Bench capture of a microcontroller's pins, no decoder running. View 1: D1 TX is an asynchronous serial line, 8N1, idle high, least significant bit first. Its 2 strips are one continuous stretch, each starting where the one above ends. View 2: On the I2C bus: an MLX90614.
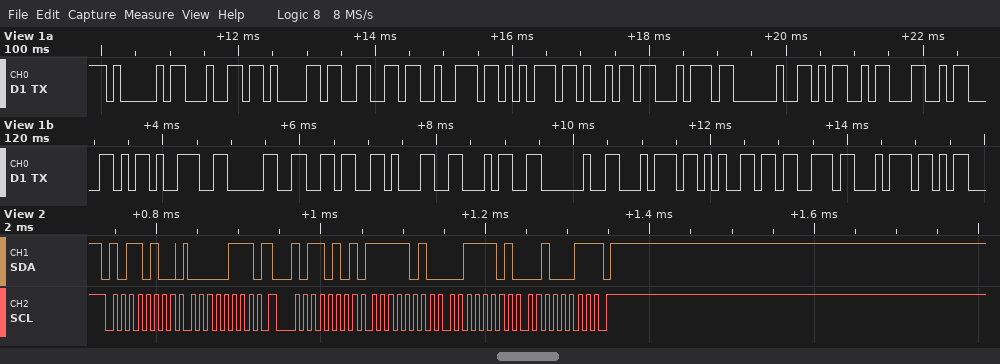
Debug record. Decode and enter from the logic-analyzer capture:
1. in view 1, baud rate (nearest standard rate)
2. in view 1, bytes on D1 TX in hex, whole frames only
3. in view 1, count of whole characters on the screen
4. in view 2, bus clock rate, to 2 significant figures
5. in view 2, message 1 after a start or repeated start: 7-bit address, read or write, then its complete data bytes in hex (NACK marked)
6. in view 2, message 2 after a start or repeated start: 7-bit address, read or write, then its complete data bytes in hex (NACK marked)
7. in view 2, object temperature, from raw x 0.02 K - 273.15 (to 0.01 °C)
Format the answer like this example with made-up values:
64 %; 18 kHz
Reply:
9600 baud; 41 64 61 66 72 75 69 74 20 4D 4C 58 39 30 36 31 34 20 74 65 73 74; 22; 100 kHz; 0x5A write: 07; 0x5A read: FA 3D 23 NACK; 44.17 °C
